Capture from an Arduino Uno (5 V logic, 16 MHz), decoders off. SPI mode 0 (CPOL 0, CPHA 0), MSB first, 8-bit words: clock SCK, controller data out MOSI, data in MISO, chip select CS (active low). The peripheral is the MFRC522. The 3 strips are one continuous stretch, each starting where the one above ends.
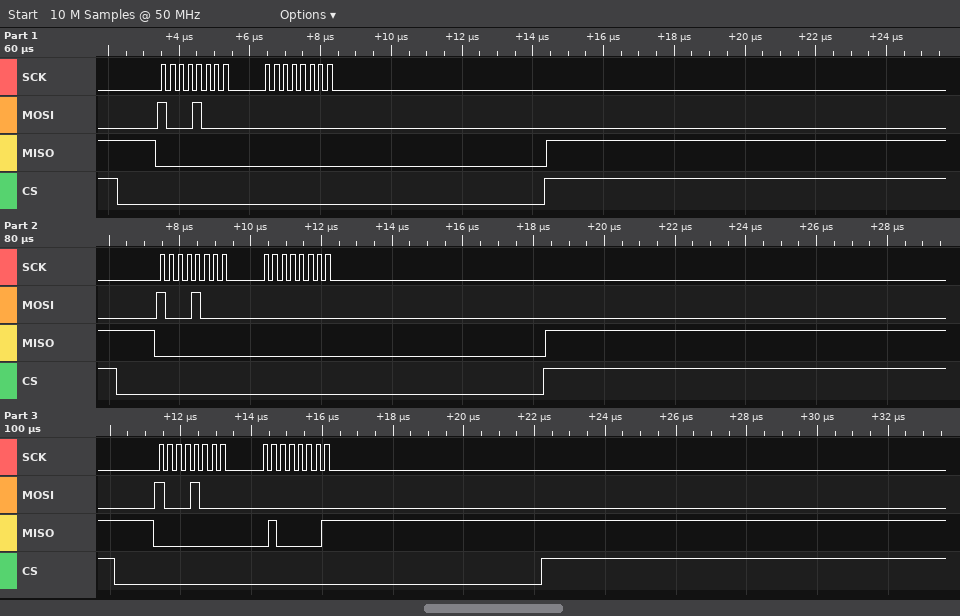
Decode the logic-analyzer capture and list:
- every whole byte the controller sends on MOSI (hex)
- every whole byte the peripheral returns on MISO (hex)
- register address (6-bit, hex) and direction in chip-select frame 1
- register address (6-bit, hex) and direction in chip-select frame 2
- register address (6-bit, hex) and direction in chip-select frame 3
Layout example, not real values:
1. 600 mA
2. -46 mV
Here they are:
1. 0x88 0x00 0x88 0x00 0x88 0x00
2. 0x00 0x00 0x00 0x00 0x00 0x41
3. 0x04 read
4. 0x04 read
5. 0x04 read
